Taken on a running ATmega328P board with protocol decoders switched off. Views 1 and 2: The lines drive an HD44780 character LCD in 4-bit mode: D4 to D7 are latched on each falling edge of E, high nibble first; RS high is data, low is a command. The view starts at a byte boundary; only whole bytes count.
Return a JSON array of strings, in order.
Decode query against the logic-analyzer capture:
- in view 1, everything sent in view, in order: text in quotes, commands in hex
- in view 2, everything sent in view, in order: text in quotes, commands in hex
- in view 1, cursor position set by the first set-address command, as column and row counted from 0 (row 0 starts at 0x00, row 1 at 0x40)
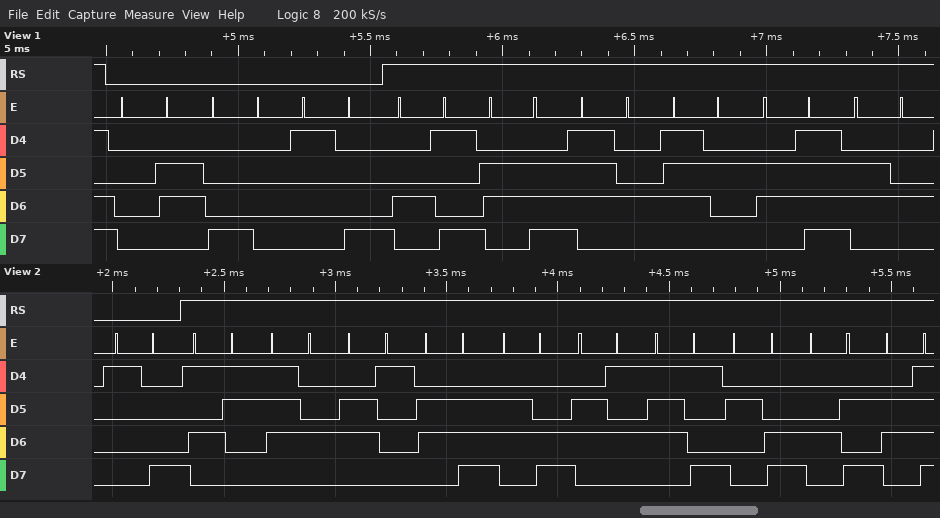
["0x06 0x80 0x18 \"Introd\"", "0x18 \"Stanley,Jo\"", "column 0, row 0"]
